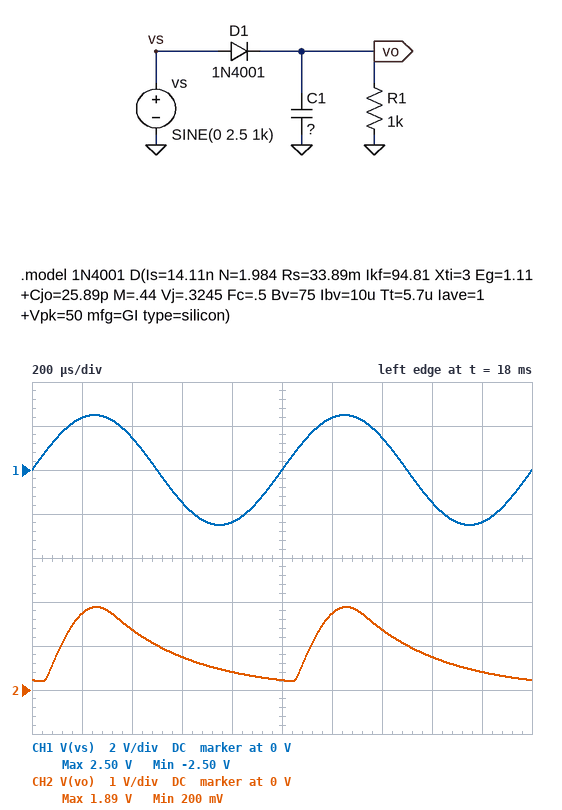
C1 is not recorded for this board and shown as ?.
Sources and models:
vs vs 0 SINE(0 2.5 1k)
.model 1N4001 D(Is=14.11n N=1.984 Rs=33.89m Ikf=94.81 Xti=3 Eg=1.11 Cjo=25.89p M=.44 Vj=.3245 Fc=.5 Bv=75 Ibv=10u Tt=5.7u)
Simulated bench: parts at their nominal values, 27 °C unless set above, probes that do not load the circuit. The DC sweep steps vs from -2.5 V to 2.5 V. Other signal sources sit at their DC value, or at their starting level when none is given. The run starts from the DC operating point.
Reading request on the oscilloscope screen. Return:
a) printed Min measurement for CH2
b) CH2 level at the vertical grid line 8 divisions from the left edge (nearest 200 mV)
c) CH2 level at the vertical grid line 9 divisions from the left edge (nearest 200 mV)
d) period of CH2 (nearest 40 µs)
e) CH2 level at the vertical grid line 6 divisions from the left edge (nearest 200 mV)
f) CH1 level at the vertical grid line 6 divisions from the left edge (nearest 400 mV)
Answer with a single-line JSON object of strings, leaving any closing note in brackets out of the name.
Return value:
{"printed Min measurement for CH2": "200 mV", "CH2 level at the vertical grid line 8 divisions from the left edge": "800 mV", "CH2 level at the vertical grid line 9 divisions from the left edge": "400 mV", "period of CH2": "1.00 ms", "CH2 level at the vertical grid line 6 divisions from the left edge": "1.8 V", "CH1 level at the vertical grid line 6 divisions from the left edge": "2.4 V"}
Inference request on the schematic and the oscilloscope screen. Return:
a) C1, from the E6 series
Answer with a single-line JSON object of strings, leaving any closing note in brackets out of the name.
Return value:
{"C1, from the E6 series": "330 nF"}
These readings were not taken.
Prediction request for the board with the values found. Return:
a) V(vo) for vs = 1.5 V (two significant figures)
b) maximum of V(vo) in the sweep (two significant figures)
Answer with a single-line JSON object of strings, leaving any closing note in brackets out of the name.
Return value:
{"V(vo) for vs = 1.5 V": "930 mV", "maximum of V(vo) in the sweep": "1.9 V"}
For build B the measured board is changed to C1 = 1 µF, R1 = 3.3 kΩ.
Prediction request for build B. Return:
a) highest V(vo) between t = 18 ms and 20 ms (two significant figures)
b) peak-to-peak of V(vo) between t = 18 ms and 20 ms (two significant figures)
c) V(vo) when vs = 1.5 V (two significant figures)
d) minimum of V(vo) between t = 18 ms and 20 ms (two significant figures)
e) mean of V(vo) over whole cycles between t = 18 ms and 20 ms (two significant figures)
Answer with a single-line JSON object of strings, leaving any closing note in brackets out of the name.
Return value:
{"highest V(vo) between t = 18 ms and 20 ms": "1.9 V", "peak-to-peak of V(vo) between t = 18 ms and 20 ms": "430 mV", "V(vo) when vs = 1.5 V": "990 mV", "minimum of V(vo) between t = 18 ms and 20 ms": "1.5 V", "mean of V(vo) over whole cycles between t = 18 ms and 20 ms": "1.7 V"}
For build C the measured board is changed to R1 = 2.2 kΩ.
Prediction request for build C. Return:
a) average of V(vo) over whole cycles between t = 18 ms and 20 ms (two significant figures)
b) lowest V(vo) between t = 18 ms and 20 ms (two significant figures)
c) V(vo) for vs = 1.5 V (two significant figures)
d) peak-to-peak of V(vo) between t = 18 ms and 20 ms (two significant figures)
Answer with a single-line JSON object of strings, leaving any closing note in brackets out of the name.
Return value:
{"average of V(vo) over whole cycles between t = 18 ms and 20 ms": "1.2 V", "lowest V(vo) between t = 18 ms and 20 ms": "650 mV", "V(vo) for vs = 1.5 V": "970 mV", "peak-to-peak of V(vo) between t = 18 ms and 20 ms": "1.3 V"}
